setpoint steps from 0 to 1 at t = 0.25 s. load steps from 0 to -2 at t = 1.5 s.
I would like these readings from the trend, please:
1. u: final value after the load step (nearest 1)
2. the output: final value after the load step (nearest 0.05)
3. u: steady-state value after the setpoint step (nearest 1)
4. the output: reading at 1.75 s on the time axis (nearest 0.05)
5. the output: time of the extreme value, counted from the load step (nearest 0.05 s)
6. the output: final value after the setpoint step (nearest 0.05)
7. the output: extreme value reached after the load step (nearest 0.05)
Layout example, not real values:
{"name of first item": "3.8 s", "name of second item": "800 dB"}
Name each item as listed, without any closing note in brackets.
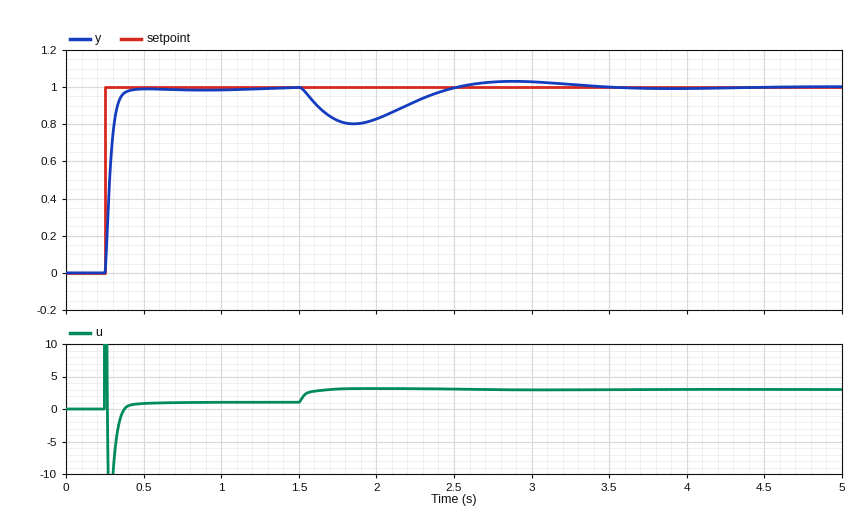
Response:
{"u: final value after the load step": "3", "the output: final value after the load step": "1.00", "u: steady-state value after the setpoint step": "1", "the output: reading at 1.75 s on the time axis": "0.80", "the output: time of the extreme value, counted from the load step": "0.35 s", "the output: final value after the setpoint step": "1.00", "the output: extreme value reached after the load step": "0.80"}
